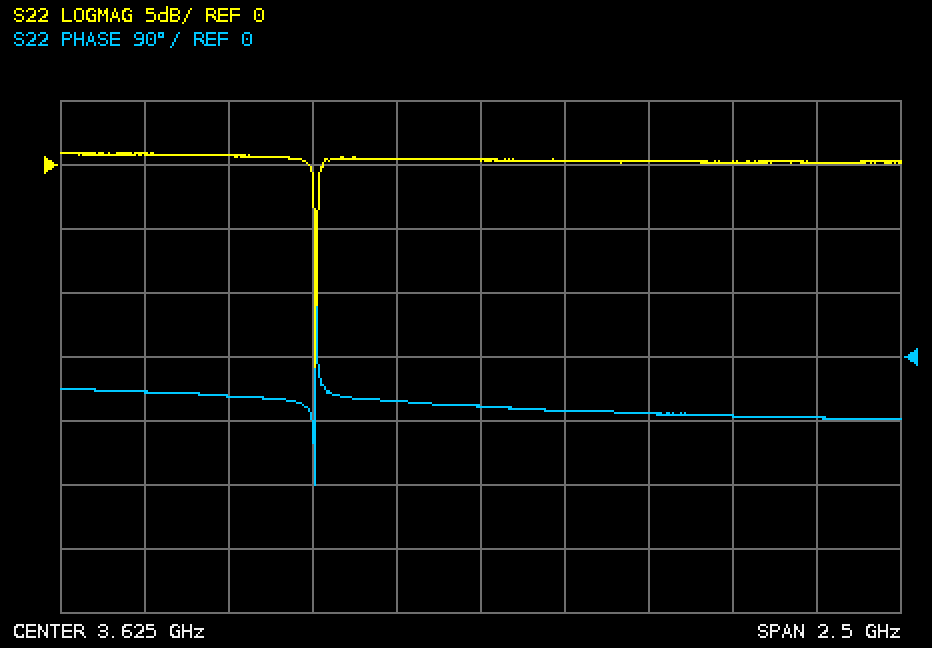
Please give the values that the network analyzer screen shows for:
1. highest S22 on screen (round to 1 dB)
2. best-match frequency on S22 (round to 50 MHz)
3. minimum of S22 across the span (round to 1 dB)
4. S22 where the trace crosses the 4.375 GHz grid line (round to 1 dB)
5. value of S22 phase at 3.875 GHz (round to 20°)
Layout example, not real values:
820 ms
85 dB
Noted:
1 dB
3.15 GHz
-16 dB
0 dB
-80°
